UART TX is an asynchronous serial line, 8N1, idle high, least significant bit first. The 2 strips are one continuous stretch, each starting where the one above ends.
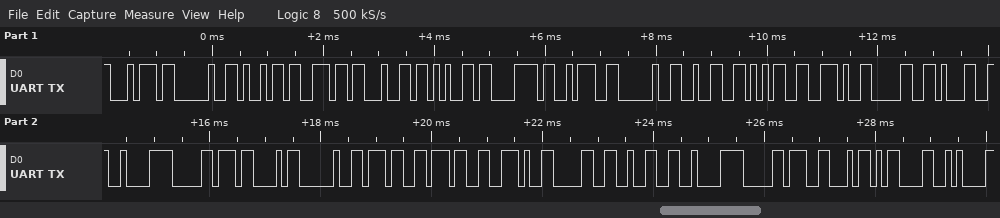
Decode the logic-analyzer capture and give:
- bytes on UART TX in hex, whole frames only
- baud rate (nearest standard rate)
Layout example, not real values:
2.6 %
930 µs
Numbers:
74 20 69 6E 64 65 78 3A 20 32 35 2E 30 31 C2 B0 43 20 37 37 2E 30 32 C2 B0 46 0D 0A
9600 baud
